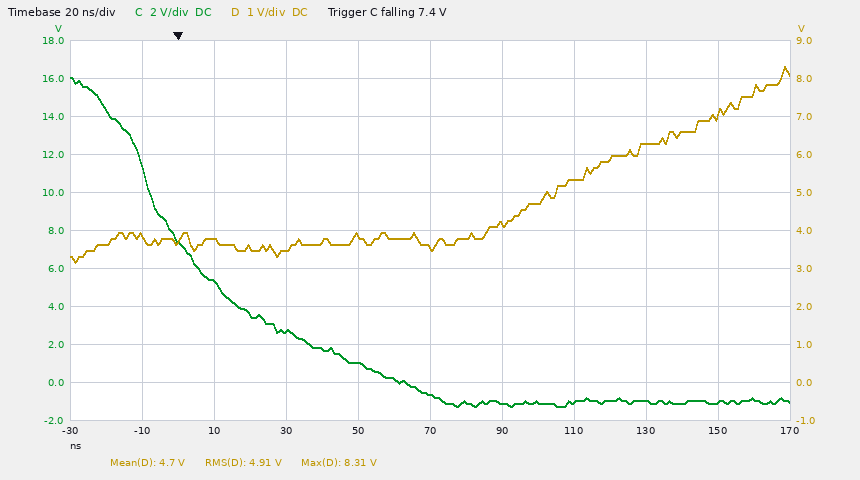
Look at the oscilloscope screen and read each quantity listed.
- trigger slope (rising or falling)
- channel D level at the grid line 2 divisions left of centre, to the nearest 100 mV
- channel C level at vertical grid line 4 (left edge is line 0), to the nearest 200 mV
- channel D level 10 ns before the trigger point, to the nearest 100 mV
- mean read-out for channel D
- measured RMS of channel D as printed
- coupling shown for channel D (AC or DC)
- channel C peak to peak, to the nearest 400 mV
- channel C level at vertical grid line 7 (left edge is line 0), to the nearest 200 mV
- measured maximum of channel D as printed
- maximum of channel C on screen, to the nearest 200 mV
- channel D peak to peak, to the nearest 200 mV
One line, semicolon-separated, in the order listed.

falling; 3.5 V; 1.0 V; 3.8 V; 4.7 V; 4.91 V; DC; 17.2 V; -1.0 V; 8.31 V; 16.0 V; 5.2 V
